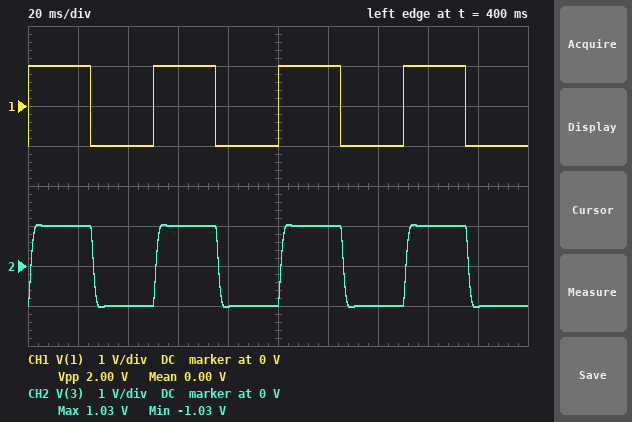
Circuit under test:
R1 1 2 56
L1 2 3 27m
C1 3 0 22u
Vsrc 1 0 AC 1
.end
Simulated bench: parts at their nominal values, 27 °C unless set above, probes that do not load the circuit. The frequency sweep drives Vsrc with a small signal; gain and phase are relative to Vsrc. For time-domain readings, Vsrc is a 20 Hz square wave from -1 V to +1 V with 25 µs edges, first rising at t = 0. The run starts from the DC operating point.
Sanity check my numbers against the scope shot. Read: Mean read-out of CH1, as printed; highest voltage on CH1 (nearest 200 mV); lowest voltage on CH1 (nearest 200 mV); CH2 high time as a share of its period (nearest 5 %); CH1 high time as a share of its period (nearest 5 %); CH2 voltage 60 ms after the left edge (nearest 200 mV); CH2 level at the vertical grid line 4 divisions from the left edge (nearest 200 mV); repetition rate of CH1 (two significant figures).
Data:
0.00 V
1.0 V
-1.0 V
50 %
50 %
1.0 V
-1.0 V
20 Hz
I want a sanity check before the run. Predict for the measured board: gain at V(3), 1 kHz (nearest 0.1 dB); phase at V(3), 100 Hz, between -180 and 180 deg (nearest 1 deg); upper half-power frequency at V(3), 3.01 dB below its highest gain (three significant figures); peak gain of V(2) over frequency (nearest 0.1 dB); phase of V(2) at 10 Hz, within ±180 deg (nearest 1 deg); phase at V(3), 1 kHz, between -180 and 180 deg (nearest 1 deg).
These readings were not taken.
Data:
-27.5 dB
-45 deg
180 Hz
0 dB
-4 deg
-161 deg
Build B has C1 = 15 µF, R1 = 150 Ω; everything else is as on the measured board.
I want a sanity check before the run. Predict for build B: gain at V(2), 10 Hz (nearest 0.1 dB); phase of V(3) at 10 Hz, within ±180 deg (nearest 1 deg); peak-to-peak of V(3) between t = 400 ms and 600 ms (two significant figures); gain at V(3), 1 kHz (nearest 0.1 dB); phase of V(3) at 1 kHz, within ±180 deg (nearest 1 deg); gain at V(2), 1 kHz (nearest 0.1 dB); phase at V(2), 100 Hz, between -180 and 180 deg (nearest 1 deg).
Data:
-0.1 dB
-8 deg
2.0 V
-26.3 dB
-137 deg
-2.8 dB
-59 deg
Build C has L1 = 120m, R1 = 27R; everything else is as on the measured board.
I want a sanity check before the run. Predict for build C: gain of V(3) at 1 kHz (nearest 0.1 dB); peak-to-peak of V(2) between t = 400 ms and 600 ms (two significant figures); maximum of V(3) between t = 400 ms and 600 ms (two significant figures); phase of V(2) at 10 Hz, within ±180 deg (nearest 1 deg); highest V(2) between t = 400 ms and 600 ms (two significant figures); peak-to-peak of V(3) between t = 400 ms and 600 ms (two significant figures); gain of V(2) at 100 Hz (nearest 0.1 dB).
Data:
-40.3 dB
2.7 V
2.2 V
-2 deg
1.3 V
4.3 V
-19.0 dB
